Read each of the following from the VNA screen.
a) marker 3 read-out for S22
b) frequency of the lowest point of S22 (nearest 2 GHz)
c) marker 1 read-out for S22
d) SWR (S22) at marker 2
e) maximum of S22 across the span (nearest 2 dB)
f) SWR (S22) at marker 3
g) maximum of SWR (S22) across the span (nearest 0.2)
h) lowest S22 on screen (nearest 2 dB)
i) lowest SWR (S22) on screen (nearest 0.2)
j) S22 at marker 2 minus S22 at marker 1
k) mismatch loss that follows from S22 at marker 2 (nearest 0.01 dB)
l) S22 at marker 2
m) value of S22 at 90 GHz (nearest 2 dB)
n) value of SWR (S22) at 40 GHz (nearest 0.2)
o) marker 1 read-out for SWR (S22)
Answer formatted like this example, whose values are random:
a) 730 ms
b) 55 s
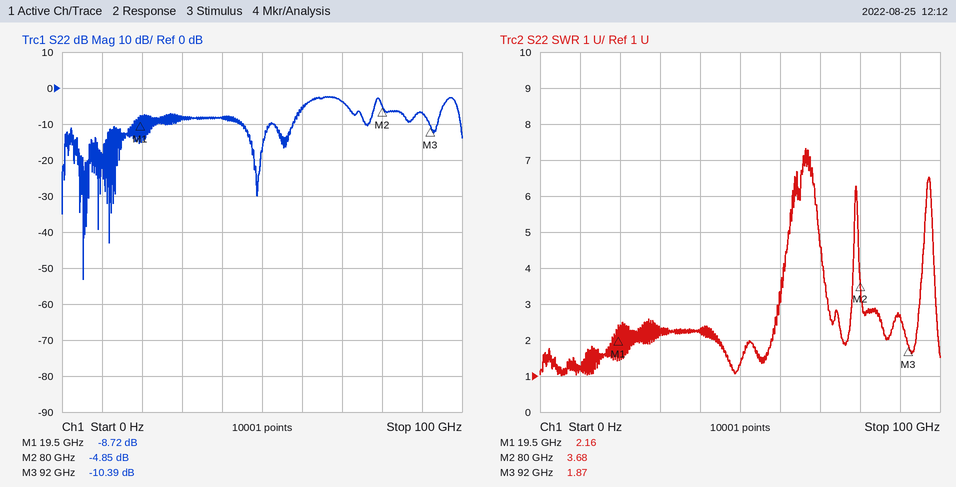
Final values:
a) -10.39 dB
b) 6 GHz
c) -8.72 dB
d) 3.68
e) -2 dB
f) 1.87
g) 7.4
h) -54 dB
i) 1.0
j) 3.87 dB
k) 1.72 dB
l) -4.85 dB
m) -6 dB
n) 2.2
o) 2.16
